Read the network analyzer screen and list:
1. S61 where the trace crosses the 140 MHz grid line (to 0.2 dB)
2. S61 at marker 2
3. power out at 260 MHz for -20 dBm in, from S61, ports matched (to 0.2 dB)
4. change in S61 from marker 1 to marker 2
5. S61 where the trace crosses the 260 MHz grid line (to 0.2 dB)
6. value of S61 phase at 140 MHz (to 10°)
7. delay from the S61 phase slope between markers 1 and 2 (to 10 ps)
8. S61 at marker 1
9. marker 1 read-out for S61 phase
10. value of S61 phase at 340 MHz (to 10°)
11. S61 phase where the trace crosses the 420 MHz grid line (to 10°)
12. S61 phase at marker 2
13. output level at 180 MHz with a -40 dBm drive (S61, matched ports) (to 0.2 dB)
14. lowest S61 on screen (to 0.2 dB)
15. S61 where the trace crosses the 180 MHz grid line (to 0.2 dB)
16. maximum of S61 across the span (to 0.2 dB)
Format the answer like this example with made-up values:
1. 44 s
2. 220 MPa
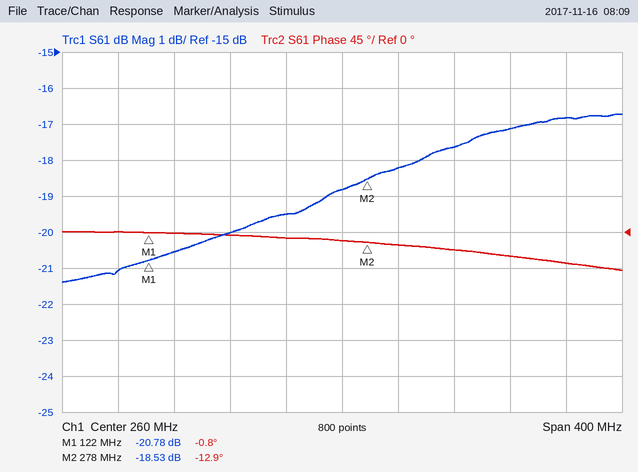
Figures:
1. -20.6 dB
2. -18.53 dB
3. -38.8 dBm
4. 2.25 dB
5. -18.8 dB
6. 0°
7. 220 ps
8. -20.78 dB
9. -0.8°
10. -20°
11. -40°
12. -12.9°
13. -60.0 dBm
14. -21.4 dB
15. -20.0 dB
16. -16.8 dB
